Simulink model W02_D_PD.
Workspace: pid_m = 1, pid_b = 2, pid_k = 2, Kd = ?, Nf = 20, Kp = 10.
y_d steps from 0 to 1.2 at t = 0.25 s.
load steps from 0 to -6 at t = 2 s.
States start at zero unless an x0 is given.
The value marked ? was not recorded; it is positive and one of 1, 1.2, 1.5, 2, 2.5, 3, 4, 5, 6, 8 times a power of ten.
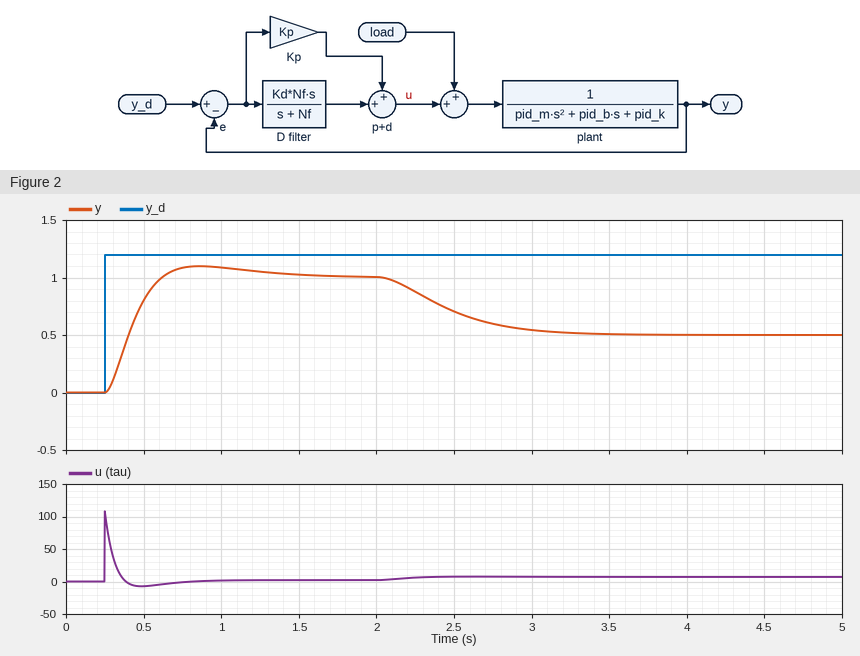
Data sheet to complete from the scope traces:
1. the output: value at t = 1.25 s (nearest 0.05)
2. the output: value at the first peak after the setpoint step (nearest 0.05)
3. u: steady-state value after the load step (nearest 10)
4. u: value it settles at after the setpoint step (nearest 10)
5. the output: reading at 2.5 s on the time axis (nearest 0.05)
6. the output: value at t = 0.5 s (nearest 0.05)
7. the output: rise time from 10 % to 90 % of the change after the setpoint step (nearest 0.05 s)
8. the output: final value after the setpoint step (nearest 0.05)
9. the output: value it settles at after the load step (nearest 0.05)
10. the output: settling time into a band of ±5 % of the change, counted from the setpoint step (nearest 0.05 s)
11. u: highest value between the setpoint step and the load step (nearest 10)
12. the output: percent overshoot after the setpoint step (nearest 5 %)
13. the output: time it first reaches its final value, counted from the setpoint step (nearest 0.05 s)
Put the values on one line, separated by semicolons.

1.05; 1.10; 10; 0; 0.70; 0.80; 0.25 s; 1.00; 0.50; 1.00 s; 110; 10 %; 0.35 s
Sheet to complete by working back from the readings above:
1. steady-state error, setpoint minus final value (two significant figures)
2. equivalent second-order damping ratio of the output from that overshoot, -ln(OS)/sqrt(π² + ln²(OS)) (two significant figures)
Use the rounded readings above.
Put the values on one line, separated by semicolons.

0.20; 0.59
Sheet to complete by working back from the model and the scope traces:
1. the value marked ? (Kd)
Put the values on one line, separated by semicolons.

4
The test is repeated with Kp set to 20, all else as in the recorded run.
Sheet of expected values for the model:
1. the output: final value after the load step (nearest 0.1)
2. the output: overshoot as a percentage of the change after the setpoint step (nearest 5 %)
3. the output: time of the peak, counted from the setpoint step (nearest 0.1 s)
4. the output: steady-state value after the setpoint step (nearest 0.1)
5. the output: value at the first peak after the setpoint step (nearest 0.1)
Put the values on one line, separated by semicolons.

0.8; 20 %; 0.5 s; 1.1; 1.3
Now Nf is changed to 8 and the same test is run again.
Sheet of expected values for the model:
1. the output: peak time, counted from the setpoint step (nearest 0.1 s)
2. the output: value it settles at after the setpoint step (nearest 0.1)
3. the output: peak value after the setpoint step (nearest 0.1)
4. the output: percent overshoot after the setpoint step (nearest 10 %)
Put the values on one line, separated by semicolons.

0.6 s; 1.0; 1.2; 20 %
